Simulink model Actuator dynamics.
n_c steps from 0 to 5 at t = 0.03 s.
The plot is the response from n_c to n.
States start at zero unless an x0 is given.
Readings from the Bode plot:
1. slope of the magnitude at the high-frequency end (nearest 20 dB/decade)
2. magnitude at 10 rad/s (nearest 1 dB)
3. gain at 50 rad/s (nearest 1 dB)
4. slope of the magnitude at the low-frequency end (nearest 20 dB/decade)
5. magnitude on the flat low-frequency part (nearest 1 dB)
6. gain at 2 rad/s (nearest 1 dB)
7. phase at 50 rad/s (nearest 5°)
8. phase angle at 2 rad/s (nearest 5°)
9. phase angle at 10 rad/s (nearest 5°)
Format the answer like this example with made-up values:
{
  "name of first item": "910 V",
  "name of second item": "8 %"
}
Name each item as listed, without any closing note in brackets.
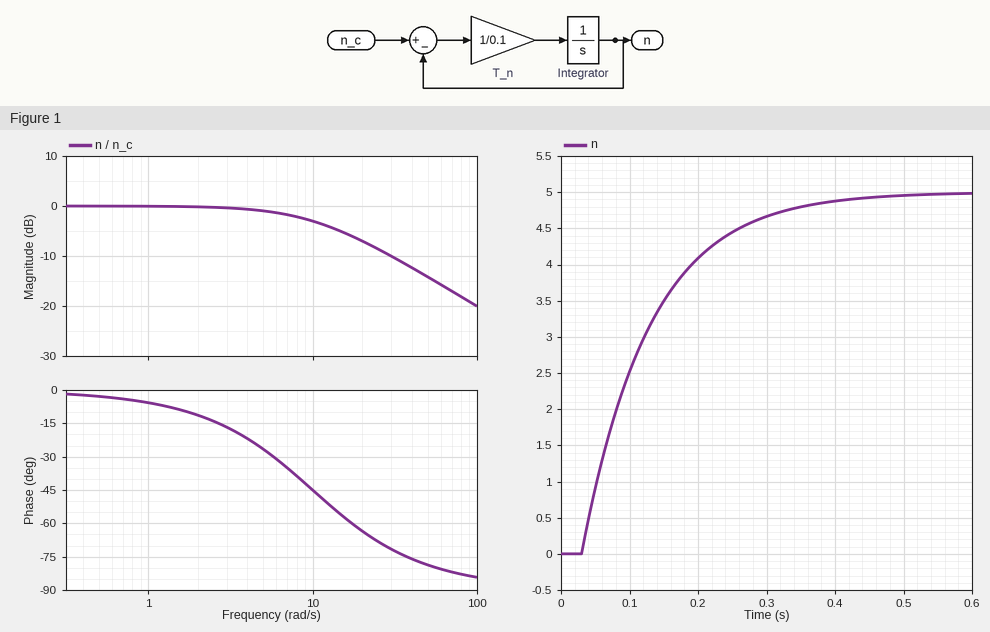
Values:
{
  "slope of the magnitude at the high-frequency end": "-20 dB/decade",
  "magnitude at 10 rad/s": "-3 dB",
  "gain at 50 rad/s": "-14 dB",
  "slope of the magnitude at the low-frequency end": "0 dB/decade",
  "magnitude on the flat low-frequency part": "0 dB",
  "gain at 2 rad/s": "0 dB",
  "phase at 50 rad/s": "-80°",
  "phase angle at 2 rad/s": "-10°",
  "phase angle at 10 rad/s": "-45°"
}
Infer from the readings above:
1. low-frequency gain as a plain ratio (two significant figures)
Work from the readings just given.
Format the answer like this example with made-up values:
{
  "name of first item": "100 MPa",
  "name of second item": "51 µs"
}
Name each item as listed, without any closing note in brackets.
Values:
{
  "low-frequency gain as a plain ratio": "1.0"
}
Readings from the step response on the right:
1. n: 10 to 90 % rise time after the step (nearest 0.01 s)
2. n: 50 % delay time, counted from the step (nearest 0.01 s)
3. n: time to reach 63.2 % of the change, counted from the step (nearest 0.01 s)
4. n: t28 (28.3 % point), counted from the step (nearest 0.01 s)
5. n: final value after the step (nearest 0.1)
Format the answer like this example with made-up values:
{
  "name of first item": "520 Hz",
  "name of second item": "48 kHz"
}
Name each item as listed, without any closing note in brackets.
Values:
{
  "n: 10 to 90 % rise time after the step": "0.22 s",
  "n: 50 % delay time, counted from the step": "0.07 s",
  "n: time to reach 63.2 % of the change, counted from the step": "0.10 s",
  "n: t28 (28.3 % point), counted from the step": "0.03 s",
  "n: final value after the step": "5.0"
}
